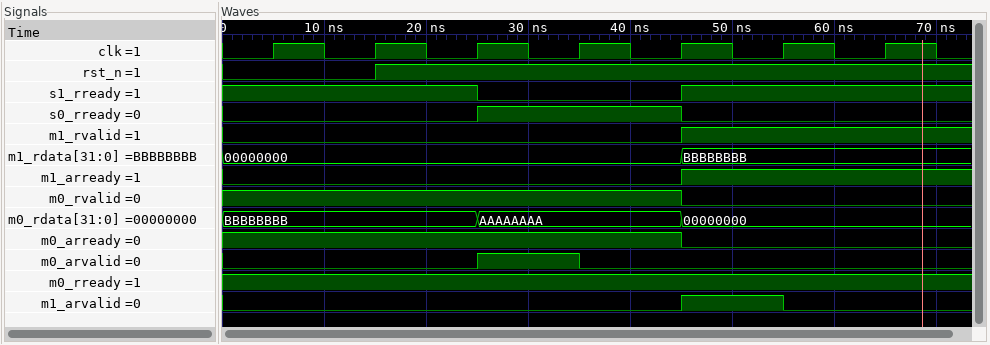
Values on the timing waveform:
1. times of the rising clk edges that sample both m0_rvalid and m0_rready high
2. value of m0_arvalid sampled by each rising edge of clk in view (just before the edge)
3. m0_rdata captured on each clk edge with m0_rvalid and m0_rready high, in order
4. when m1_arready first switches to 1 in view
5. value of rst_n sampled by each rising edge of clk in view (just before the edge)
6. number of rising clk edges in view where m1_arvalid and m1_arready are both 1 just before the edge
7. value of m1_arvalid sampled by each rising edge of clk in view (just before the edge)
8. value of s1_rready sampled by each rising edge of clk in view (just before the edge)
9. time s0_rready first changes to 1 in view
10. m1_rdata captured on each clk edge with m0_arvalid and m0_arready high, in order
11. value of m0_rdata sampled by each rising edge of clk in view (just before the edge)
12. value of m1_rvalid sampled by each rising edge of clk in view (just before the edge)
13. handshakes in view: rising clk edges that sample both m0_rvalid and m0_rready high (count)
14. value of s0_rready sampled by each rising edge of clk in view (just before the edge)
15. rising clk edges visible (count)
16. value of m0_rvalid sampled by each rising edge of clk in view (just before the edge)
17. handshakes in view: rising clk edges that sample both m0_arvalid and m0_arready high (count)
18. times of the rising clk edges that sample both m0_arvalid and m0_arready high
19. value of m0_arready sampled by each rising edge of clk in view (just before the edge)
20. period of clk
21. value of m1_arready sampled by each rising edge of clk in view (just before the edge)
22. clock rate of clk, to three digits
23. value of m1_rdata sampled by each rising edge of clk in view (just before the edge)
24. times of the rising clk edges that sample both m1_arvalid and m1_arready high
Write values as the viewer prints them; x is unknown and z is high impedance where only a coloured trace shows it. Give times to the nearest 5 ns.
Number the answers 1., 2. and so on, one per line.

1. 5 ns, 15 ns, 25 ns, 35 ns, 45 ns
2. 0 0 0 1 0 0 0
3. BBBBBBBB, BBBBBBBB, BBBBBBBB, AAAAAAAA, AAAAAAAA
4. 45 ns
5. 0 0 1 1 1 1 1
6. 1
7. 0 0 0 0 0 1 0
8. 1 1 1 0 0 1 1
9. 25 ns
10. 00000000
11. BBBBBBBB, BBBBBBBB, BBBBBBBB, AAAAAAAA, AAAAAAAA, 00000000, 00000000
12. 0 0 0 0 0 1 1
13. 5
14. 0 0 0 1 1 0 0
15. 7
16. 1 1 1 1 1 0 0
17. 1
18. 35 ns
19. 1 1 1 1 1 0 0
20. 10 ns
21. 0 0 0 0 0 1 1
22. 100 MHz
23. 00000000, 00000000, 00000000, 00000000, 00000000, BBBBBBBB, BBBBBBBB
24. 55 ns
